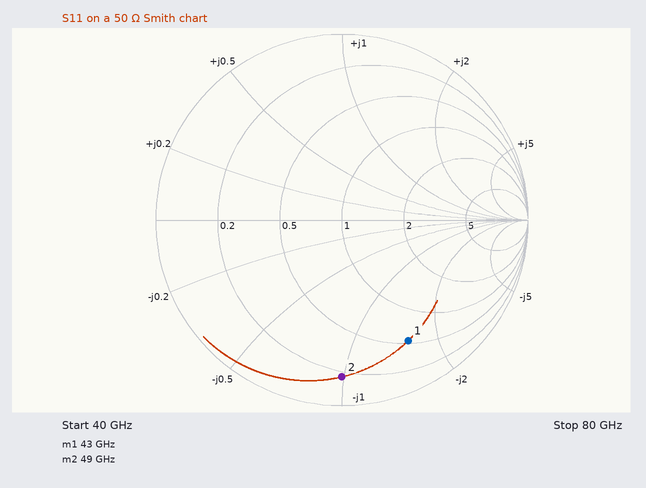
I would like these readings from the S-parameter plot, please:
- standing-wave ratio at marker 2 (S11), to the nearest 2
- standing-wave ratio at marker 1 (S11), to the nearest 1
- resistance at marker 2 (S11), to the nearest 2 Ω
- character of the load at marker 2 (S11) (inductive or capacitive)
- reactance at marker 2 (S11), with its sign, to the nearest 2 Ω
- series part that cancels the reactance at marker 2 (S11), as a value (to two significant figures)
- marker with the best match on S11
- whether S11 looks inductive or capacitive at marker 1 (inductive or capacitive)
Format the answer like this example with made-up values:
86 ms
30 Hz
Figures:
12
7
8 Ω
capacitive
-50 Ω
160 pH
marker 1
capacitive
